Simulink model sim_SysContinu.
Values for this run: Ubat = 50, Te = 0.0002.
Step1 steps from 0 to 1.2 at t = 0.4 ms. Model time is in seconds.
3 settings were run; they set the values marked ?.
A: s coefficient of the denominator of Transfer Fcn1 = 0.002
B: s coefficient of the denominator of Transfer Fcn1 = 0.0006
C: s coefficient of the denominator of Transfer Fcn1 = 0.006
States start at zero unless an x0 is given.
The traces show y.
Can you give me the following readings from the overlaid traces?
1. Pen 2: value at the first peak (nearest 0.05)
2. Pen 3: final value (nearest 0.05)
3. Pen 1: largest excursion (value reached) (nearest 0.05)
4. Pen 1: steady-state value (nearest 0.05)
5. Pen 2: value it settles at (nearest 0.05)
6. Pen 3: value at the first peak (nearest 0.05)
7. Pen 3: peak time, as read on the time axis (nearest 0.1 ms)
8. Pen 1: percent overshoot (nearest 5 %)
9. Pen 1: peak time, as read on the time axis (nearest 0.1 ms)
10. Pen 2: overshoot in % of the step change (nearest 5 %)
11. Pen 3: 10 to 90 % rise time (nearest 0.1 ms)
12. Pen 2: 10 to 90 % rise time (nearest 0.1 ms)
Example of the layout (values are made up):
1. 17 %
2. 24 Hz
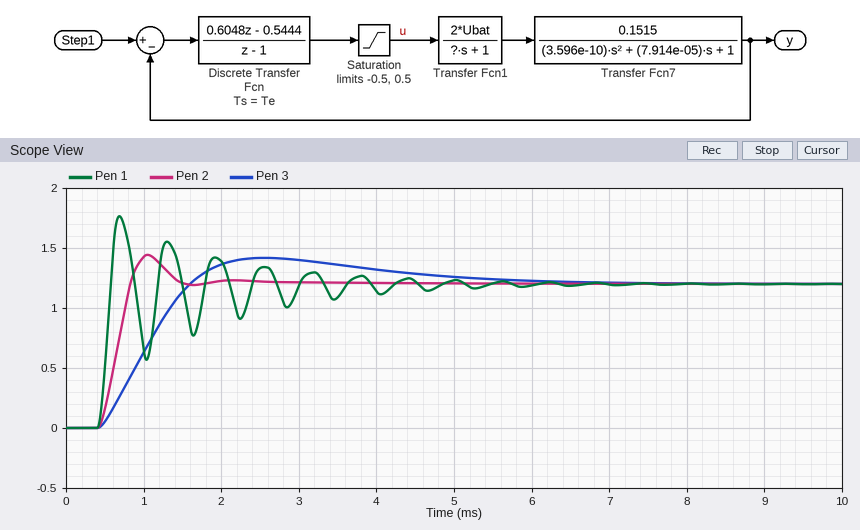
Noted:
1. 1.45
2. 1.20
3. 1.75
4. 1.20
5. 1.20
6. 1.40
7. 2.6 ms
8. 45 %
9. 0.7 ms
10. 20 %
11. 0.9 ms
12. 0.3 ms
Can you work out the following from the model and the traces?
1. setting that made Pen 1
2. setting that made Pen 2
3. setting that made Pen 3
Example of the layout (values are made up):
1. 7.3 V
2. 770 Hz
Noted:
1. B
2. A
3. C
